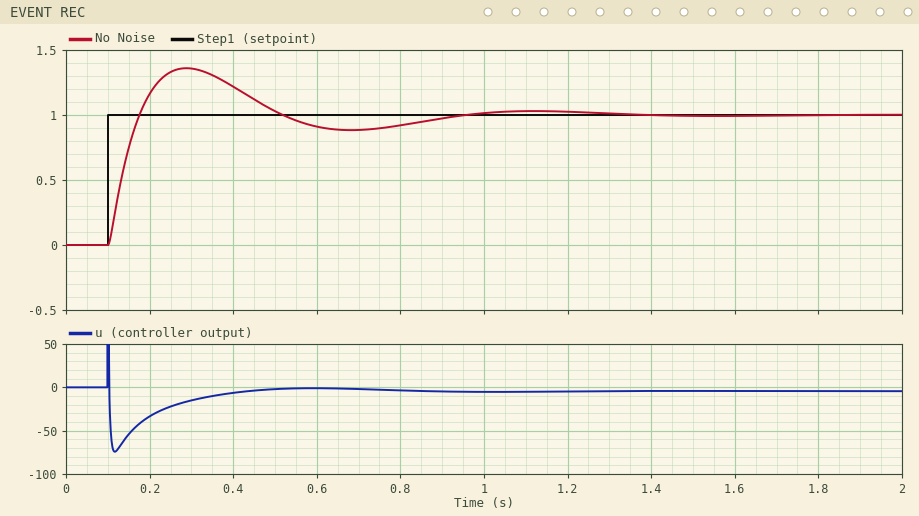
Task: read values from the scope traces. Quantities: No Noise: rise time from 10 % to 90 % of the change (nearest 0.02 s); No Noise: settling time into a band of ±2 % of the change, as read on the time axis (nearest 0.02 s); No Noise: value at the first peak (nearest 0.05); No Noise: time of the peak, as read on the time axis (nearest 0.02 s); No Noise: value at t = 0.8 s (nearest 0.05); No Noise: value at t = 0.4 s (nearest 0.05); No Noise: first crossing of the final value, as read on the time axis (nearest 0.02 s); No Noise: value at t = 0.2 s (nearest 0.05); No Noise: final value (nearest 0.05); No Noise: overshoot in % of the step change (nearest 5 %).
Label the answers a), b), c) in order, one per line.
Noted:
a) 0.06 s
b) 1.24 s
c) 1.35
d) 0.28 s
e) 0.90
f) 1.20
g) 0.18 s
h) 1.15
i) 1.00
j) 35 %
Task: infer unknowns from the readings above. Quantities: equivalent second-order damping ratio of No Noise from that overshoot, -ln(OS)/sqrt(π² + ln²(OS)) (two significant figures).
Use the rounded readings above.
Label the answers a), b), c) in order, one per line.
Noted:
a) 0.32
